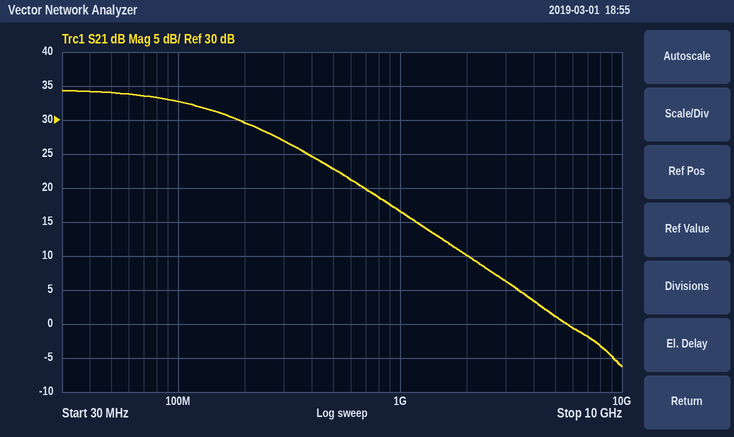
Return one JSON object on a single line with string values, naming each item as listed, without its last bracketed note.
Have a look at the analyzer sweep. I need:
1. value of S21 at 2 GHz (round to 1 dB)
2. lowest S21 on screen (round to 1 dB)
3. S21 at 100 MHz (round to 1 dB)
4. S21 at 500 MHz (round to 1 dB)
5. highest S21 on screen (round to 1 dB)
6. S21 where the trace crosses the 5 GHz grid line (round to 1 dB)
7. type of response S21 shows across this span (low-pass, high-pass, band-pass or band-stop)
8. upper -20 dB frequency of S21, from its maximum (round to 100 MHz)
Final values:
{"value of S21 at 2 GHz": "10 dB", "lowest S21 on screen": "-6 dB", "S21 at 100 MHz": "33 dB", "S21 at 500 MHz": "23 dB", "highest S21 on screen": "34 dB", "S21 where the trace crosses the 5 GHz grid line": "1 dB", "type of response S21 shows across this span": "low-pass", "upper -20 dB frequency of S21, from its maximum": "1.3 GHz"}
